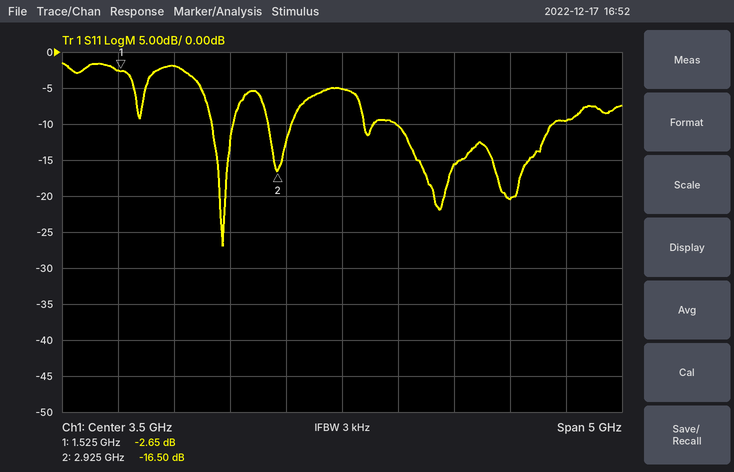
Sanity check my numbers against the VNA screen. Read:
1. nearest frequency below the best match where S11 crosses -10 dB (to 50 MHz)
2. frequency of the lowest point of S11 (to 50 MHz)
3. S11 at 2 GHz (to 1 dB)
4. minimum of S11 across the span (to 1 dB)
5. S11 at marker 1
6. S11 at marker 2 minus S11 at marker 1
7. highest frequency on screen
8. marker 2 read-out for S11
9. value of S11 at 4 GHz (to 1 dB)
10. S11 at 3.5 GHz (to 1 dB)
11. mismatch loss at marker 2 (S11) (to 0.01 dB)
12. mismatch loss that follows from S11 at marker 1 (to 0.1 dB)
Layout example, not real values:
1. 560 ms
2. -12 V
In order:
1. 2.35 GHz
2. 2.45 GHz
3. -2 dB
4. -27 dB
5. -2.65 dB
6. -13.85 dB
7. 6 GHz
8. -16.50 dB
9. -10 dB
10. -5 dB
11. 0.10 dB
12. 3.4 dB
